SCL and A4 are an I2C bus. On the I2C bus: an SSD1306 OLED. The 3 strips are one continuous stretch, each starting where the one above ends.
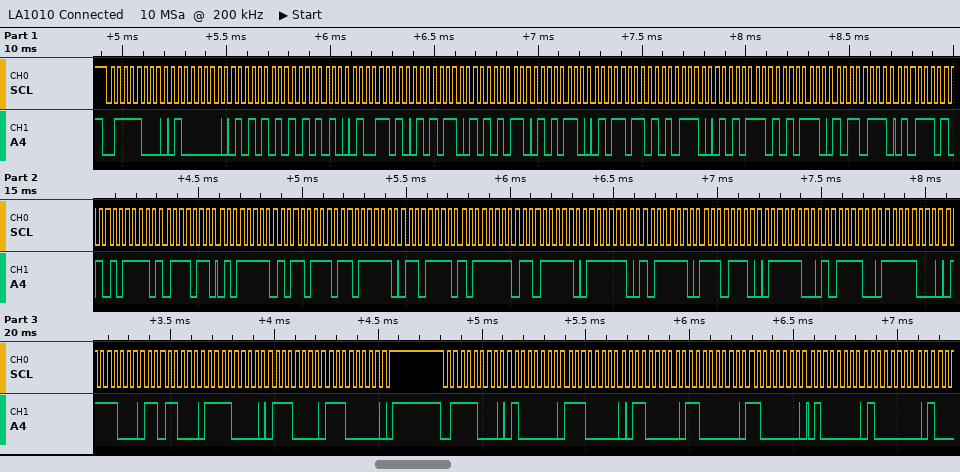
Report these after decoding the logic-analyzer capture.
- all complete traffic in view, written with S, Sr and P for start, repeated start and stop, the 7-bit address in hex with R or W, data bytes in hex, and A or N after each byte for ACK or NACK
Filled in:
S 3CW A 40 A 55 A AA A 4D A 56 A AB A 56 A 5B A AE A 57 A AE A B7 A 5D A AF A BB A 5F A B7 A DF A 6F A BF A DF A 7E A BE A EE A 7C A BC A F8 A 78 A D8 A F0 A 70 A E0 A P S 3CW A 40 A E0 A 60 A C0 A C0 A 40 A 80 A
